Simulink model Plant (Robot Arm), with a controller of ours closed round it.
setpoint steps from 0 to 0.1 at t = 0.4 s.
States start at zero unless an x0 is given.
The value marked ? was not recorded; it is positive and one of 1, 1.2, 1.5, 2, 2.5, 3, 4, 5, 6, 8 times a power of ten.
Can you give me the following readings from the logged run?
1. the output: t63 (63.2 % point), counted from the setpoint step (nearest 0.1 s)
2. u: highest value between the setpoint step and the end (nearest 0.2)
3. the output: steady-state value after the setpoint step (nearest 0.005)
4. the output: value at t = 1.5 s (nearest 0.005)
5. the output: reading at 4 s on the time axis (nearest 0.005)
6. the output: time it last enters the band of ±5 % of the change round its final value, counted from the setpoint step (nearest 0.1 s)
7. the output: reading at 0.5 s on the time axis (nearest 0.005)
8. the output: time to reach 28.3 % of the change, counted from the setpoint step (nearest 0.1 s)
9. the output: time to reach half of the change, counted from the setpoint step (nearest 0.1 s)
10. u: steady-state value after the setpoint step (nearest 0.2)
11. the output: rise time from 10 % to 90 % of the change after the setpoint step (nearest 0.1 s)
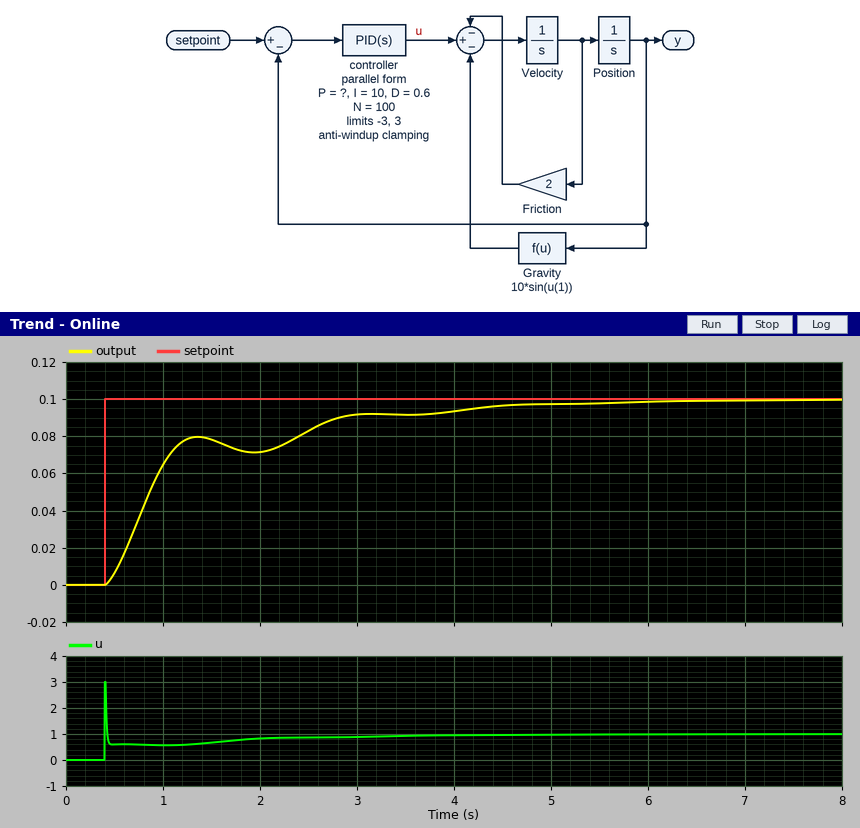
0.6 s
3.0
0.100
0.080
0.095
3.8 s
0.005
0.3 s
0.5 s
1.0
2.3 s
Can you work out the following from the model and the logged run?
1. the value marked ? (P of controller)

6
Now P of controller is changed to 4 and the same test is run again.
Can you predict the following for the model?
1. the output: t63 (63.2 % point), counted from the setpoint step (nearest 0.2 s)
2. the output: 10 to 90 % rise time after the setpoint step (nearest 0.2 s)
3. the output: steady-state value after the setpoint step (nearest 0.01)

0.8 s
2.4 s
0.10
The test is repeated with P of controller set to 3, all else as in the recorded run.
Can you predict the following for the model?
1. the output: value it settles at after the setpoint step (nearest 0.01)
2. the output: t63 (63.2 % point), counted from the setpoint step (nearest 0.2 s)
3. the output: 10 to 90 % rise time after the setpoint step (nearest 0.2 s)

0.10
0.8 s
2.4 s
